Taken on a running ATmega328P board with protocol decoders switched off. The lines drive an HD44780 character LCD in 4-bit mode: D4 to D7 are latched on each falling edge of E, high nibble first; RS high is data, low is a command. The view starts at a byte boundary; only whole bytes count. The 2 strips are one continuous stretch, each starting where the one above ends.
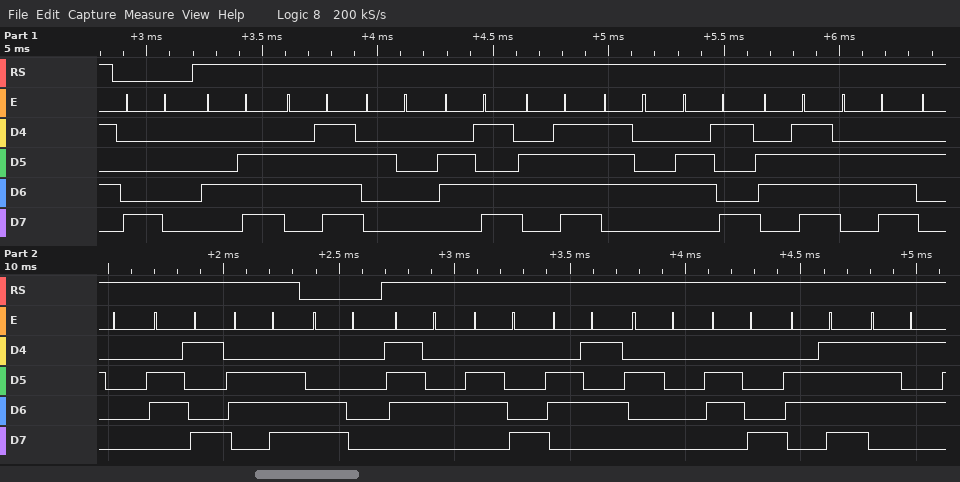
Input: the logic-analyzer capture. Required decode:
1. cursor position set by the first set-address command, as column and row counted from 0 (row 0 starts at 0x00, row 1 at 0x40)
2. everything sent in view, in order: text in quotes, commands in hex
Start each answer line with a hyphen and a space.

- column 0, row 0
- 0x80 "No motion in" 0xC0 "the hou"
